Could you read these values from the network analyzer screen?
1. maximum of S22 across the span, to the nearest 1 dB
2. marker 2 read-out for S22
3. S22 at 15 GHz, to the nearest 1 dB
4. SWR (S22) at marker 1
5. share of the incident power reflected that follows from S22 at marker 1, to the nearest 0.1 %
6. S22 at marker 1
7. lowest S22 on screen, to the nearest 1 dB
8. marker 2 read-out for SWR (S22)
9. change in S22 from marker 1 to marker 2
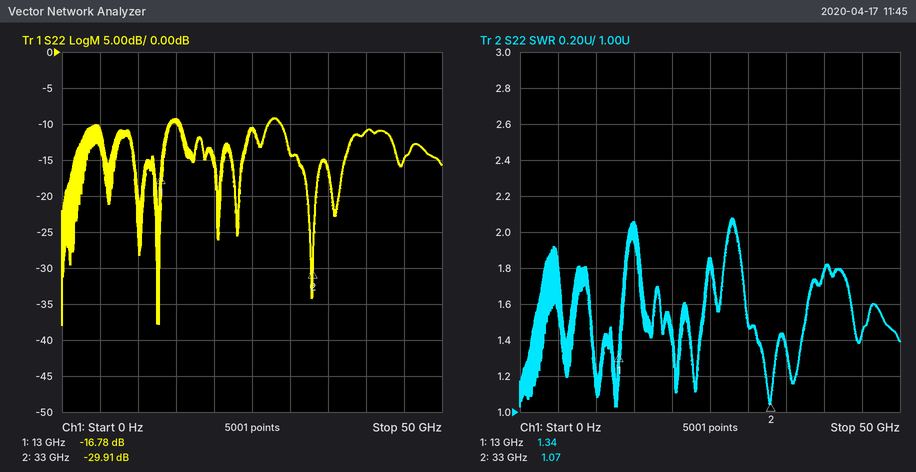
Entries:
-9 dB
-29.91 dB
-10 dB
1.34
2.1 %
-16.78 dB
-38 dB
1.07
-13.13 dB
